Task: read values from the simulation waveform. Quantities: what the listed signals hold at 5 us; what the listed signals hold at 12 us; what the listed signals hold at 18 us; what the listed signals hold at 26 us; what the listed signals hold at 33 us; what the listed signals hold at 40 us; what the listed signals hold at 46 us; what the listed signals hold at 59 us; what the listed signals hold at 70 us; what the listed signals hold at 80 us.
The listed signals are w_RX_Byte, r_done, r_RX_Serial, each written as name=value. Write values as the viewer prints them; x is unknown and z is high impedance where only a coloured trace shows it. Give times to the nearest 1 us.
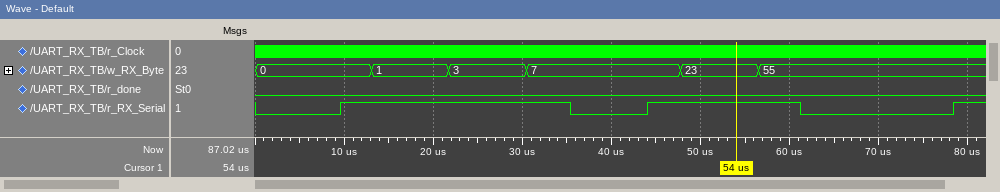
w_RX_Byte=0, r_done=0, r_RX_Serial=0
w_RX_Byte=0, r_done=0, r_RX_Serial=1
w_RX_Byte=1, r_done=0, r_RX_Serial=1
w_RX_Byte=3, r_done=0, r_RX_Serial=1
w_RX_Byte=7, r_done=0, r_RX_Serial=1
w_RX_Byte=7, r_done=0, r_RX_Serial=0
w_RX_Byte=7, r_done=0, r_RX_Serial=1
w_RX_Byte=55, r_done=0, r_RX_Serial=1
w_RX_Byte=55, r_done=0, r_RX_Serial=0
w_RX_Byte=55, r_done=0, r_RX_Serial=1
